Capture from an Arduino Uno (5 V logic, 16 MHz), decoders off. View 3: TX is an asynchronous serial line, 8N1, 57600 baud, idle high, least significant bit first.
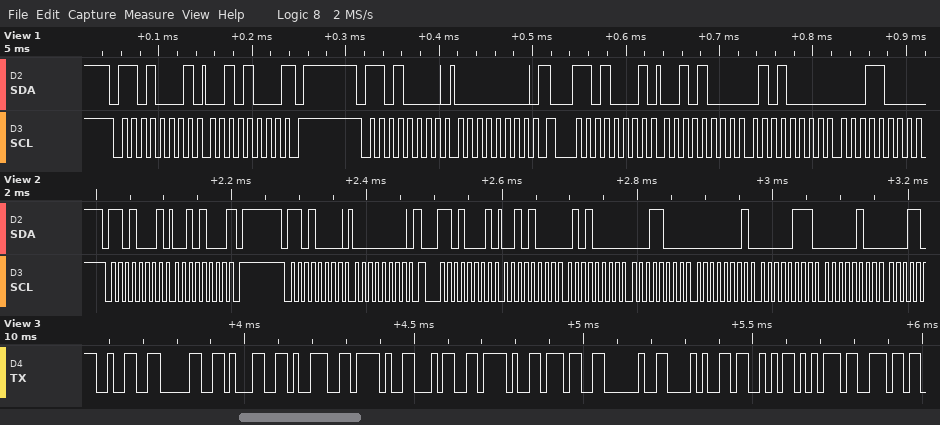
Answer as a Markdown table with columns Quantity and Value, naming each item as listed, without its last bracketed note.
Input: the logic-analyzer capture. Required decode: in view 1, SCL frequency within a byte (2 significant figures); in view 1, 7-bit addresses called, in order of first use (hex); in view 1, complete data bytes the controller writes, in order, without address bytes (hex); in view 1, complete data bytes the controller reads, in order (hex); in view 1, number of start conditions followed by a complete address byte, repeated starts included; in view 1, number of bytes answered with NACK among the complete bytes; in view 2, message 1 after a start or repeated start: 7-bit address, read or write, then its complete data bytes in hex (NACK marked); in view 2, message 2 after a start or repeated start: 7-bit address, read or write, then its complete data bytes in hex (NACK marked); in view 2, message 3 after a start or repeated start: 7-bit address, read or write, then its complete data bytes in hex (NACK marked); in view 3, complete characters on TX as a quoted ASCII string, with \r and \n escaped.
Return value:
| Quantity | Value |
|---|---|
| in view 1, SCL frequency within a byte | 100 kHz |
| in view 1, 7-bit addresses called, in order of first use | 0x68 |
| in view 1, complete data bytes the controller writes, in order, without address bytes | 00 |
| in view 1, complete data bytes the controller reads, in order | 28 28 50 18 |
| in view 1, number of start conditions followed by a complete address byte, repeated starts included | 3 |
| in view 1, number of bytes answered with NACK among the complete bytes | 1 |
| in view 2, message 1 after a start or repeated start: 7-bit address, read or write, then its complete data bytes in hex | 0x68 read: 28 NACK |
| in view 2, message 2 after a start or repeated start: 7-bit address, read or write, then its complete data bytes in hex | 0x68 write: 00 |
| in view 2, message 3 after a start or repeated start: 7-bit address, read or write, then its complete data bytes in hex | 0x68 read: 28 50 18 01 07 04 |
| in view 3, complete characters on TX as a quoted ASCII string, with \r and \n escaped | "2019/4/7 (Sun" |
